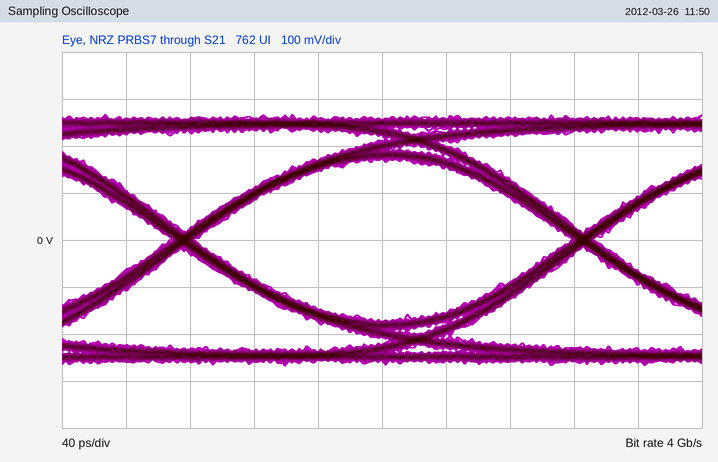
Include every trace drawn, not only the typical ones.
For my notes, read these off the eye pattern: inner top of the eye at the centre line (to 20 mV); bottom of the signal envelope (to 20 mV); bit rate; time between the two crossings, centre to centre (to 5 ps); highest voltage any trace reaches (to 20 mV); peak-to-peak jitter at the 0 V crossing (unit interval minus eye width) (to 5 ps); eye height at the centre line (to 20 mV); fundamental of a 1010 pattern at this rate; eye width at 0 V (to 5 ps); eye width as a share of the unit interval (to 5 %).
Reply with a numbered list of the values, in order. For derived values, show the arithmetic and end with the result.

1. 180 mV
2. -260 mV
3. 4 Gb/s
4. 250 ps
5. 260 mV
6. 15 ps
7. 340 mV
8. 2 GHz
9. 235 ps
10. 235 ps / 250 ps ≈ 94.0 %, so 95 % to the nearest 5 %
